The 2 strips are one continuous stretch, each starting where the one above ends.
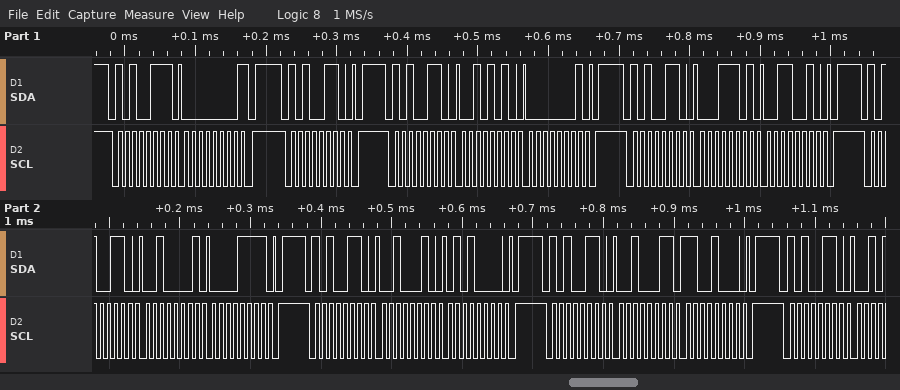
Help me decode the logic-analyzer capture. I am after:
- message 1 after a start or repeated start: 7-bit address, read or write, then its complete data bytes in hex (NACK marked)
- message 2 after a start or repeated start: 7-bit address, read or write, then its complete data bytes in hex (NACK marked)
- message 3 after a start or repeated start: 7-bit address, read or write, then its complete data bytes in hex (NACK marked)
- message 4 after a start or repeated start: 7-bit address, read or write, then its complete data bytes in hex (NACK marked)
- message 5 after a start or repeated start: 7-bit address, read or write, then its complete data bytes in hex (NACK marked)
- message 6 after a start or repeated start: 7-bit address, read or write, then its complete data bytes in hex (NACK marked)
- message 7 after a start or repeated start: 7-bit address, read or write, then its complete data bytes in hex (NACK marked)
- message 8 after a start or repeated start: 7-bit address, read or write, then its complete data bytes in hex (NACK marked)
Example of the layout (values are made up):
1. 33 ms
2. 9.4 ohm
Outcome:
1. 0x53 read: 00 NACK
2. 0x53 write
3. 0x53 write: 2A 01
4. 0x53 write: 1D 32
5. 0x53 write: 21 0F
6. 0x53 write: 22 50
7. 0x53 write: 23 C8
8. 0x53 write
